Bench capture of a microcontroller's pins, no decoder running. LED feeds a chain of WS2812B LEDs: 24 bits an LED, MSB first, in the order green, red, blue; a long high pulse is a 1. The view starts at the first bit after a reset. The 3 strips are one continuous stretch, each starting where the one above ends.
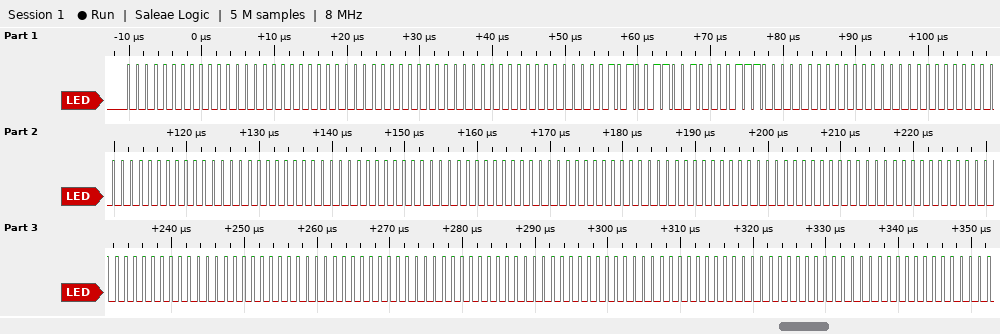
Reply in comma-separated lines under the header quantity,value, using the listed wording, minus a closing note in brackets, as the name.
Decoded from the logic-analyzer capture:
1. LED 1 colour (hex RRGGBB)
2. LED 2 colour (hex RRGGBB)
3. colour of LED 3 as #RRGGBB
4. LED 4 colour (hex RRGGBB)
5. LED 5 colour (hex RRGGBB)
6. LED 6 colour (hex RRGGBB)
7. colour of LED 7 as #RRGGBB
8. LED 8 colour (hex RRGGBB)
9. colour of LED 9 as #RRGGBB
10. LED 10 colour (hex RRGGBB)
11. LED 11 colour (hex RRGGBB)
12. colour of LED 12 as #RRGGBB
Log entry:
quantity,value
LED 1 colour,#000000
LED 2 colour,#000000
colour of LED 3 as #RRGGBB,#32051C
LED 4 colour,#000000
LED 5 colour,#000000
LED 6 colour,#000000
colour of LED 7 as #RRGGBB,#000000
LED 8 colour,#000000
colour of LED 9 as #RRGGBB,#000000
LED 10 colour,#000000
LED 11 colour,#000000
colour of LED 12 as #RRGGBB,#000000
